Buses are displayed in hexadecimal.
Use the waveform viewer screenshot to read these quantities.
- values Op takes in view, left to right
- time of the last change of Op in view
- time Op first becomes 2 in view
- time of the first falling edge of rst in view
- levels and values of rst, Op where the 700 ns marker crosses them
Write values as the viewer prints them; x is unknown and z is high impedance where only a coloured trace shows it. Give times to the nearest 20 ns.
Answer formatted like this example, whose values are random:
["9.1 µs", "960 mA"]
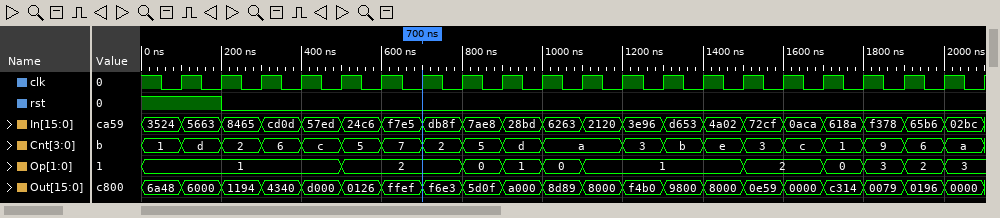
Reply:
["1, 2, 0, 1, 0, 1, 2, 0, 3, 2, 3", "2000 ns", "500 ns", "200 ns", "rst=0, Op=2"]
